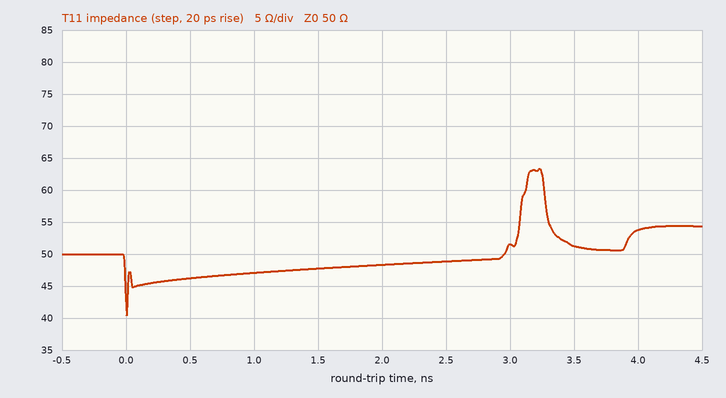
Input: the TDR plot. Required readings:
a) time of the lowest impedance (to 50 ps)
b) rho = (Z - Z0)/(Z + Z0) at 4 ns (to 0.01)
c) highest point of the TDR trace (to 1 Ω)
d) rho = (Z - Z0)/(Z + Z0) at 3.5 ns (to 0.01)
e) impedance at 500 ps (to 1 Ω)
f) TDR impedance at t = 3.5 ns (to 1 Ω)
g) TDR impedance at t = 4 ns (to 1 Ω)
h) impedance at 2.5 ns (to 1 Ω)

0 ps
+0.04
63 Ω
+0.01
46 Ω
51 Ω
54 Ω
49 Ω
